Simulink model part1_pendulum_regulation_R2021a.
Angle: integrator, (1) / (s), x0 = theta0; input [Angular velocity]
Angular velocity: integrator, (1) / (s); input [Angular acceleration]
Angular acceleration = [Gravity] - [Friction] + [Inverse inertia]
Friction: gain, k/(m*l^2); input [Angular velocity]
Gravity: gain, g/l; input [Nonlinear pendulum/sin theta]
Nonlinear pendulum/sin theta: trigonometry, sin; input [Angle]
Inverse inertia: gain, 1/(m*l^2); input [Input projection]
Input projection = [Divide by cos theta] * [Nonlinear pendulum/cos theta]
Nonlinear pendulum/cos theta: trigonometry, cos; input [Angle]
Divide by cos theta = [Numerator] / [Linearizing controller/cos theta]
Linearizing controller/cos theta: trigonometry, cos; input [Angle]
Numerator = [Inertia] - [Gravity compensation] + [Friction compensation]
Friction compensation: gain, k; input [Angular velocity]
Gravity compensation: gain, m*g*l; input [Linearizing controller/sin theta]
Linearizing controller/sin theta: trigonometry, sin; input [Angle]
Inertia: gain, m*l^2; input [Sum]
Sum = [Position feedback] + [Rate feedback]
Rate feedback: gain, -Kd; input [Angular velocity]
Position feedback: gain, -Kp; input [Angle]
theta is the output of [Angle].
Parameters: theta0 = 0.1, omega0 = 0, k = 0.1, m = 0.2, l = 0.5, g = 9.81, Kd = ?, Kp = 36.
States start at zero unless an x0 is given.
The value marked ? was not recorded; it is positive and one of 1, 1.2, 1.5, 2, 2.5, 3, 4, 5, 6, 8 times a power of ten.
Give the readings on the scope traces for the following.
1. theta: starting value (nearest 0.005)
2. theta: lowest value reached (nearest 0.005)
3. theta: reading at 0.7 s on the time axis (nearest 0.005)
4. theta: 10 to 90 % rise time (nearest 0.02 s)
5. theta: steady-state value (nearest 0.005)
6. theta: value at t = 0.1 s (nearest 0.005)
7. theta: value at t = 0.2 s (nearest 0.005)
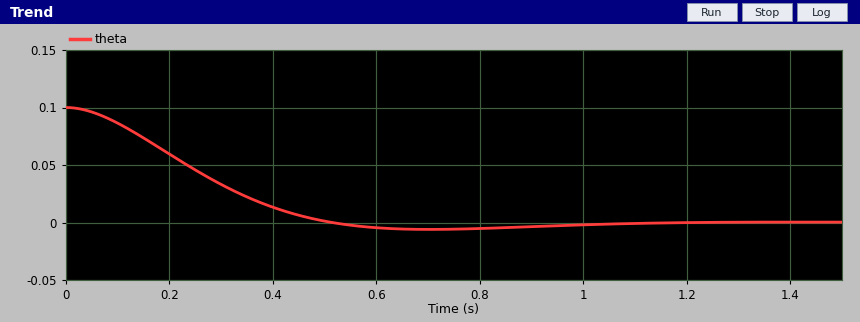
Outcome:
0.100
-0.005
-0.005
0.34 s
0.000
0.085
0.060
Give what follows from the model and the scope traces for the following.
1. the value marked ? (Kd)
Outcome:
8
